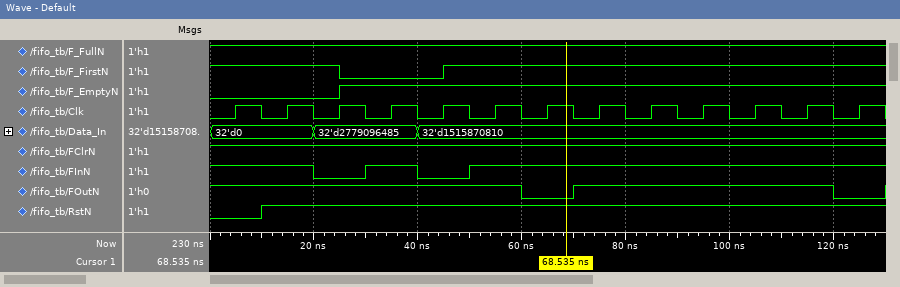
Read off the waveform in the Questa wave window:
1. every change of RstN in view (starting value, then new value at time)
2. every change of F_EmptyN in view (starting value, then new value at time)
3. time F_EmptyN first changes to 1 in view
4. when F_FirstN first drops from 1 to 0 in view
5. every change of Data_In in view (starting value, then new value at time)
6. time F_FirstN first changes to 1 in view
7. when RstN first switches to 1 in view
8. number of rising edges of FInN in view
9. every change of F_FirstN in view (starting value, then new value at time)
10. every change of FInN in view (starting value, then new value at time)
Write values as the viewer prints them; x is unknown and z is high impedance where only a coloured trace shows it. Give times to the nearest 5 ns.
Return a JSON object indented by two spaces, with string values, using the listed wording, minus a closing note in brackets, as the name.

{
  "every change of RstN in view": "0, 1 at 10 ns",
  "every change of F_EmptyN in view": "0, 1 at 25 ns",
  "time F_EmptyN first changes to 1 in view": "25 ns",
  "when F_FirstN first drops from 1 to 0 in view": "25 ns",
  "every change of Data_In in view": "32'd0, 32'd2779096485 at 20 ns, 32'd1515870810 at 40 ns",
  "time F_FirstN first changes to 1 in view": "45 ns",
  "when RstN first switches to 1 in view": "10 ns",
  "number of rising edges of FInN in view": "2",
  "every change of F_FirstN in view": "1, 0 at 25 ns, 1 at 45 ns",
  "every change of FInN in view": "1, 0 at 20 ns, 1 at 30 ns, 0 at 40 ns, 1 at 50 ns"
}
